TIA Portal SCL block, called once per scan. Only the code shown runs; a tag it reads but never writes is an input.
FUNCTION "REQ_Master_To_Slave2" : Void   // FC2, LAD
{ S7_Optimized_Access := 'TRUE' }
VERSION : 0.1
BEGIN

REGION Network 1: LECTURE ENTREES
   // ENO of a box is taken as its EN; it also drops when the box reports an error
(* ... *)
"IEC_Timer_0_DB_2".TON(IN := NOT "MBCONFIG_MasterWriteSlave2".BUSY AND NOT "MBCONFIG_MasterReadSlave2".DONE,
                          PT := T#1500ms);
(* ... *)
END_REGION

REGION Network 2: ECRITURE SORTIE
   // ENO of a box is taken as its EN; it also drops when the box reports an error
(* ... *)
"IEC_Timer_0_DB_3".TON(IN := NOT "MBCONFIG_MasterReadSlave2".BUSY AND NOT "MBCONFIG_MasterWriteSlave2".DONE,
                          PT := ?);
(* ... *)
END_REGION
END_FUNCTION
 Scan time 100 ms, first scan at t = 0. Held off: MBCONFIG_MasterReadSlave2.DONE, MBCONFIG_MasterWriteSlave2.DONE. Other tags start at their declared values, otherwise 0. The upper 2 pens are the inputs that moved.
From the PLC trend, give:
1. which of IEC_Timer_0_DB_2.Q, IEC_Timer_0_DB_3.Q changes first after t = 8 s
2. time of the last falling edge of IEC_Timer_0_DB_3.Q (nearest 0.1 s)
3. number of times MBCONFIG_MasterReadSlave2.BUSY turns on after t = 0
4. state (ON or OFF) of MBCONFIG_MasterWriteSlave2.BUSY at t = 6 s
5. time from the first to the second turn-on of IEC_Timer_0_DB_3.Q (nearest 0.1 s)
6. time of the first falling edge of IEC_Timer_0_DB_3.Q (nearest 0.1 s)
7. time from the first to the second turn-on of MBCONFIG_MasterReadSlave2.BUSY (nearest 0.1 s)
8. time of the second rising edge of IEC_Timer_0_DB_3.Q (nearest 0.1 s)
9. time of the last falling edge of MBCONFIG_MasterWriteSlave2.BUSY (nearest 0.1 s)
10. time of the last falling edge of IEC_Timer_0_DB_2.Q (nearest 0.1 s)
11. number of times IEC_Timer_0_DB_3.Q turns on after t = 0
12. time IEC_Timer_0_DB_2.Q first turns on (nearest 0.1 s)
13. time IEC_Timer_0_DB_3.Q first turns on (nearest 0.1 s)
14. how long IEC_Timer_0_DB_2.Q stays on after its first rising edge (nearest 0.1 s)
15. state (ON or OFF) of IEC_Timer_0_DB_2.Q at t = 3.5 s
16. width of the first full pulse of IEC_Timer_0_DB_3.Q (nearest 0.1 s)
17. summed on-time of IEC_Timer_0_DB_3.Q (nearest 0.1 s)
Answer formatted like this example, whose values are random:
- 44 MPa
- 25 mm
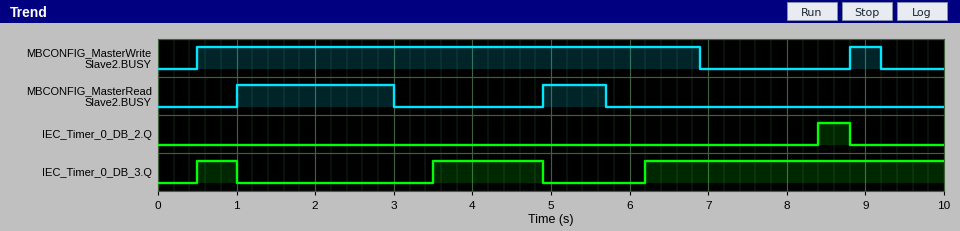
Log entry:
- IEC_Timer_0_DB_2.Q
- 4.9 s
- 2
- ON
- 3.0 s
- 1.0 s
- 3.9 s
- 3.5 s
- 9.2 s
- 8.8 s
- 3
- 8.4 s
- 0.5 s
- 0.4 s
- OFF
- 0.5 s
- 5.7 s
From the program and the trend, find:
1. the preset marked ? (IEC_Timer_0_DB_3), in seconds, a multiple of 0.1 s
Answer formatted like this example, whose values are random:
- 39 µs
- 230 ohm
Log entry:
- 0.5 s
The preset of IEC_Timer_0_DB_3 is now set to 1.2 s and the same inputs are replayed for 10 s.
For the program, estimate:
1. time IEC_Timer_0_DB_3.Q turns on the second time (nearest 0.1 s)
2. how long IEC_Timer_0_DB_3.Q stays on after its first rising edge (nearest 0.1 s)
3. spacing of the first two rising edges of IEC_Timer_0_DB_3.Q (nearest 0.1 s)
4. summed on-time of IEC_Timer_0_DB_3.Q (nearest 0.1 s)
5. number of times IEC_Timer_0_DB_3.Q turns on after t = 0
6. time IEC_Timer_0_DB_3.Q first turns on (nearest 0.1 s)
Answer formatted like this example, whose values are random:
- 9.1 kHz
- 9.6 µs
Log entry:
- 6.9 s
- 0.7 s
- 2.7 s
- 3.8 s
- 2
- 4.2 s
